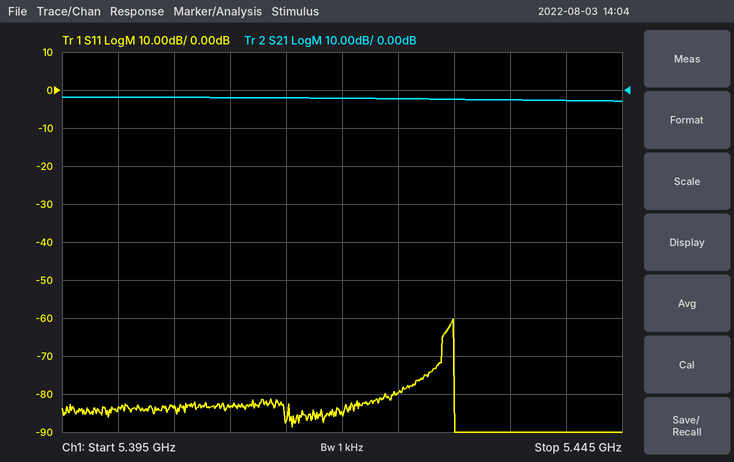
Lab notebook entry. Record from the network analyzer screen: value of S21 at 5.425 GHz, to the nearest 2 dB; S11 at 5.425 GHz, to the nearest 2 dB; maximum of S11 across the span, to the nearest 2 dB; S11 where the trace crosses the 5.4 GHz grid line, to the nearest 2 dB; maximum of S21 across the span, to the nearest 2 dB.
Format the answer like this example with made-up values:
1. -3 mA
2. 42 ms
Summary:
1. -2 dB
2. -80 dB
3. -60 dB
4. -84 dB
5. -2 dB
